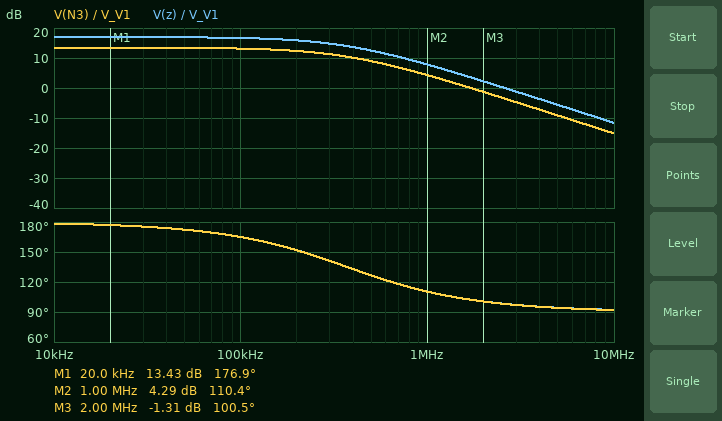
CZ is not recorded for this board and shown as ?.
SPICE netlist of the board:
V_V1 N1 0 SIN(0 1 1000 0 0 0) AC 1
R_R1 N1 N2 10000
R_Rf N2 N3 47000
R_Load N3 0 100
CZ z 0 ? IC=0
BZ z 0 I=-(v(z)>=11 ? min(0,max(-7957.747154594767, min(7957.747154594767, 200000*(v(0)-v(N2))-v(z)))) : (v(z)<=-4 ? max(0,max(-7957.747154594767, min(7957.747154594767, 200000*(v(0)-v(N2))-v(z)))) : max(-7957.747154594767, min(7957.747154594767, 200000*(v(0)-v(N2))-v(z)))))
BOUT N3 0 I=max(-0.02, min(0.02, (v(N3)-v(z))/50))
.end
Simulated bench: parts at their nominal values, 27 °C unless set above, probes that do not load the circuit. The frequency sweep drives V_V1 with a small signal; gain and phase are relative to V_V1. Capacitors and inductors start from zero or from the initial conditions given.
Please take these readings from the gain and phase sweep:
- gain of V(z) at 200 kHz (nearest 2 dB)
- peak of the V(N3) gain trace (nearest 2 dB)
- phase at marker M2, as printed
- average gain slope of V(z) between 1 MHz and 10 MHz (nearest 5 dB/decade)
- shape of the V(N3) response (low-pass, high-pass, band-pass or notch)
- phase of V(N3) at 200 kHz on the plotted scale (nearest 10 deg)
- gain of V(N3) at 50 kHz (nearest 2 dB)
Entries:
16 dB
14 dB
110.4 deg
-20 dB/decade
low-pass
150 deg
14 dB
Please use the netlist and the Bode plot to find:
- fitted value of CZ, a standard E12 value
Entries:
10 mF
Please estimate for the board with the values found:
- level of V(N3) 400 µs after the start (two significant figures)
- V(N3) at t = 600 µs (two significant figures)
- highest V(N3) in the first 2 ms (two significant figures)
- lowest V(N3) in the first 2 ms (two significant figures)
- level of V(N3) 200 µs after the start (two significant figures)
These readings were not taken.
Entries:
-2.0 V
2.0 V
2.0 V
-2.0 V
-2.0 V
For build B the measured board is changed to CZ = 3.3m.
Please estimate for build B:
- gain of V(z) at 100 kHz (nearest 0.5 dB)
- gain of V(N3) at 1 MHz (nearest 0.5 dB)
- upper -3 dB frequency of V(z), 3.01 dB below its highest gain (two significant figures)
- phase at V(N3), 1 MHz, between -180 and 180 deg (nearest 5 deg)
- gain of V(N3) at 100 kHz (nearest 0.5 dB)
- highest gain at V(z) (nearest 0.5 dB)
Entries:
17.0 dB
11.0 dB
1.1 MHz
140 deg
13.5 dB
17.0 dB
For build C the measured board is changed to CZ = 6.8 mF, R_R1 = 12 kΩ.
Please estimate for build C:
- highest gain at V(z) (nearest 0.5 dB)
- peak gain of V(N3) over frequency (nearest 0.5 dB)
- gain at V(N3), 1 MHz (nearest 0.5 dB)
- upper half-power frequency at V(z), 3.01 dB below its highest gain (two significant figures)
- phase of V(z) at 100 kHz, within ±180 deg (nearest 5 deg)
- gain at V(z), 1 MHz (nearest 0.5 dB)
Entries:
15.5 dB
12.0 dB
6.5 dB
630 kHz
170 deg
10.0 dB
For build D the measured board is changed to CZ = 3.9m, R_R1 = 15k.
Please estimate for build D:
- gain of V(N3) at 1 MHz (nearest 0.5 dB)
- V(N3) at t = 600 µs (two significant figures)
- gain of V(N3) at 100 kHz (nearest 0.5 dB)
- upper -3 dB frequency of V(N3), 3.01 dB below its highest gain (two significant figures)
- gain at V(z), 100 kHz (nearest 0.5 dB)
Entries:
8.0 dB
1.8 V
10.0 dB
1.3 MHz
13.5 dB
